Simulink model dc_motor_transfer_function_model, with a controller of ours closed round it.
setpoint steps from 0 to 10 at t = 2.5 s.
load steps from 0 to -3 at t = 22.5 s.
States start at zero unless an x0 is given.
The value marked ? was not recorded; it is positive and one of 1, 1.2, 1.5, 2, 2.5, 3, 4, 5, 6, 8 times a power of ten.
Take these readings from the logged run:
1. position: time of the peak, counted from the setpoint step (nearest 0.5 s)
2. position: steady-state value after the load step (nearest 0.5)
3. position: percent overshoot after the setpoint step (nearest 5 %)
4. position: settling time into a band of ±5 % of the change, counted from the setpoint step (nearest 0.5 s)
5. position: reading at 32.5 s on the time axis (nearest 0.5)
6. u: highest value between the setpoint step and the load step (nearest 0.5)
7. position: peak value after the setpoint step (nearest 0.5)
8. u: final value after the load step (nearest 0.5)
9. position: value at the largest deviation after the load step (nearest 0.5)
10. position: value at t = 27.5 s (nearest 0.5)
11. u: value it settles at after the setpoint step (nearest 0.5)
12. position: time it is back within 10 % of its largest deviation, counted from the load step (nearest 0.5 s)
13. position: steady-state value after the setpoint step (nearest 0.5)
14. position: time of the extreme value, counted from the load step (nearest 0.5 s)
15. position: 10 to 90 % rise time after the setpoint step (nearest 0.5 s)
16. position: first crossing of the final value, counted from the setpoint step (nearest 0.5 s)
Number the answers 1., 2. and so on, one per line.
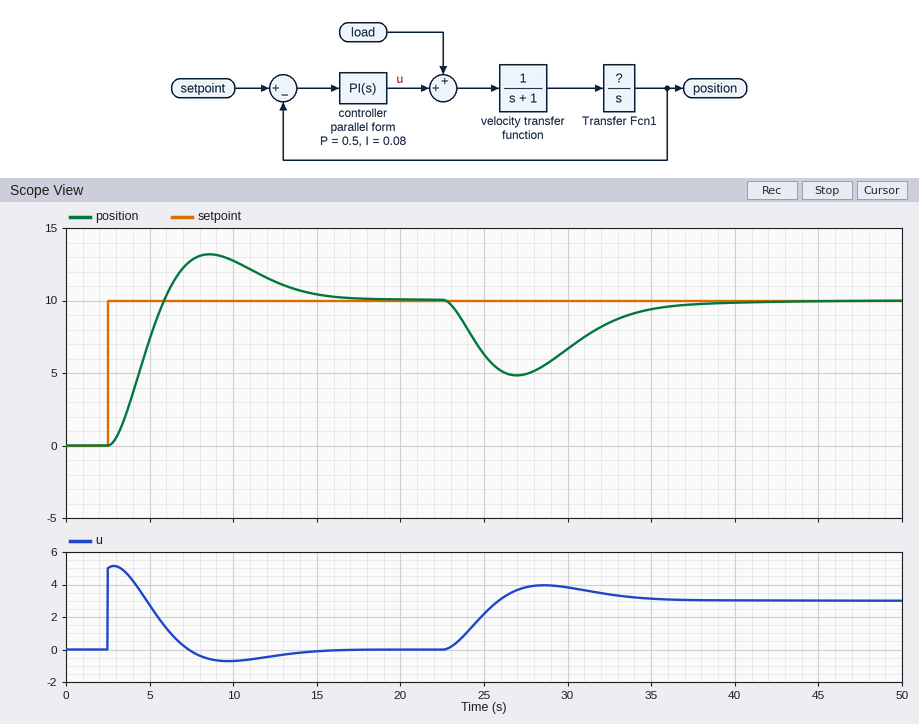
1. 6.0 s
2. 10.0
3. 30 %
4. 12.0 s
5. 8.5
6. 5.0
7. 13.0
8. 3.0
9. 5.0
10. 5.0
11. 0.0
12. 13.0 s
13. 10.0
14. 4.5 s
15. 2.5 s
16. 3.5 s
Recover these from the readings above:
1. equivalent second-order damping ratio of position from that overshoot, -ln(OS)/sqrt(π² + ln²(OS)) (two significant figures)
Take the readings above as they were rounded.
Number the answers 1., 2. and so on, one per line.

1. 0.36
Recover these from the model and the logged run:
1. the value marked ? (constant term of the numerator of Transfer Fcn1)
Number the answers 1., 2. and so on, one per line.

1. 1
